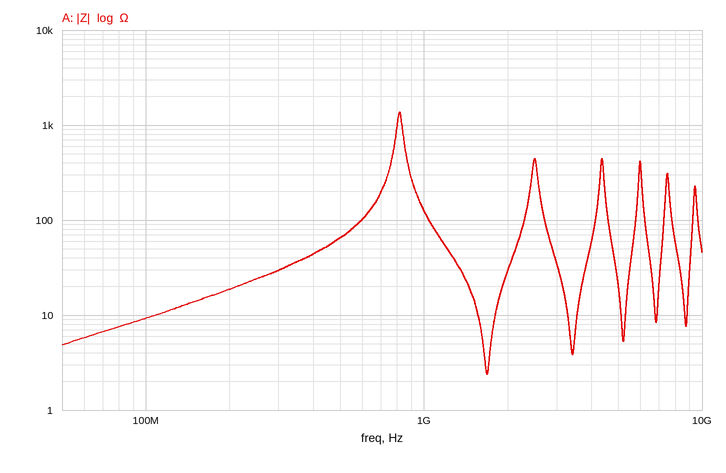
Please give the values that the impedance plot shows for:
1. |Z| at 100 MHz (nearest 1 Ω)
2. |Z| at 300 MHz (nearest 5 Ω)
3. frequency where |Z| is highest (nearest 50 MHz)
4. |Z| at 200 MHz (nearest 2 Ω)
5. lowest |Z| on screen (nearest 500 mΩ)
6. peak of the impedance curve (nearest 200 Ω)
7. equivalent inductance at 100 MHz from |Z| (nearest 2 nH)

9 Ω
30 Ω
800 MHz
18 Ω
2.5 Ω
1.4 kΩ
14 nH
